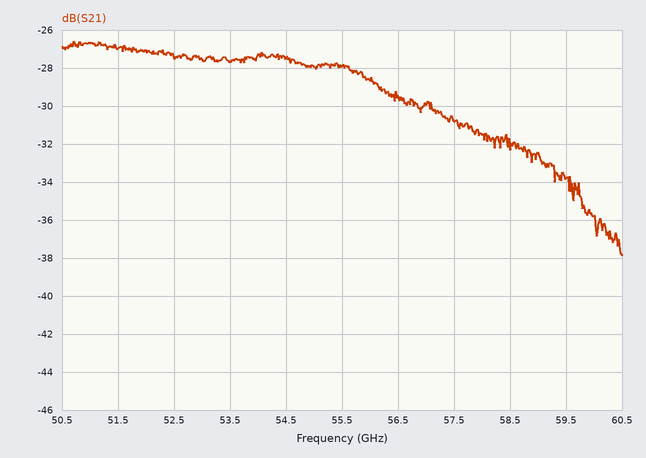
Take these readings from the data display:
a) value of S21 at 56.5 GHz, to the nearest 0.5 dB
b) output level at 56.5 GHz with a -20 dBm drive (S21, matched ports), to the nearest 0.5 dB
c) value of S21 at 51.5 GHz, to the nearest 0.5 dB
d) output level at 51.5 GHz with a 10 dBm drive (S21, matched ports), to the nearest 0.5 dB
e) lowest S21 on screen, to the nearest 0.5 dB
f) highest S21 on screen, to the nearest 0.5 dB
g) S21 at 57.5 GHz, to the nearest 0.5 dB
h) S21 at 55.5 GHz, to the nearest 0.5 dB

-29.5 dB
-49.5 dBm
-27.0 dB
-17.0 dBm
-38.0 dB
-26.5 dB
-31.0 dB
-28.0 dB
